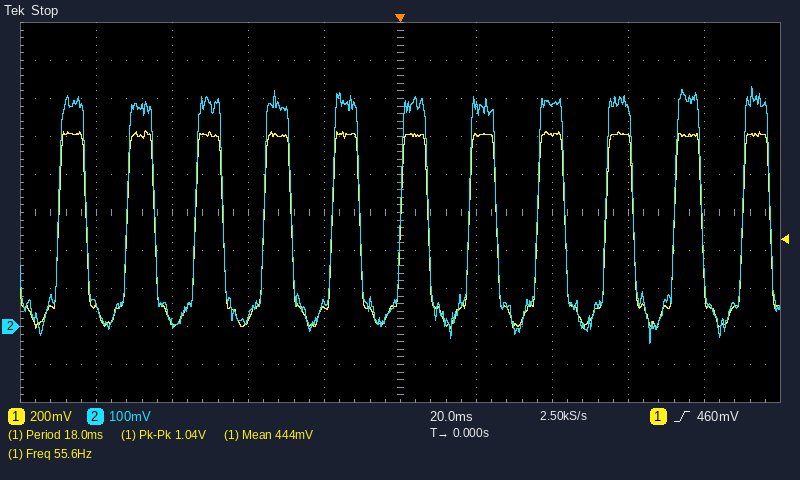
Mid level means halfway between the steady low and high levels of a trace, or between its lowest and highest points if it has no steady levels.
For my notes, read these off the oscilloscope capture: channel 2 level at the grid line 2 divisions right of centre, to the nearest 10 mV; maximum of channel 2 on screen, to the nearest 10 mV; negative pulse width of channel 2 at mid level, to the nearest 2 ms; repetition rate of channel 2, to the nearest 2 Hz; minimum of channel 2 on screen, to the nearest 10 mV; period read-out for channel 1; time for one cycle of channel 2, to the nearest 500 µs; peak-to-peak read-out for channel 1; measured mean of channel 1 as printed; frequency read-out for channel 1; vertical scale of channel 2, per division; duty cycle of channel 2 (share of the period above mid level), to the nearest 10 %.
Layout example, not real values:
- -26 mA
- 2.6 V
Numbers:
- 590 mV
- 630 mV
- 10 ms
- 56 Hz
- -40 mV
- 18.0 ms
- 18.0 ms
- 1.04 V
- 444 mV
- 55.6 Hz
- 100 mV
- 40 %
